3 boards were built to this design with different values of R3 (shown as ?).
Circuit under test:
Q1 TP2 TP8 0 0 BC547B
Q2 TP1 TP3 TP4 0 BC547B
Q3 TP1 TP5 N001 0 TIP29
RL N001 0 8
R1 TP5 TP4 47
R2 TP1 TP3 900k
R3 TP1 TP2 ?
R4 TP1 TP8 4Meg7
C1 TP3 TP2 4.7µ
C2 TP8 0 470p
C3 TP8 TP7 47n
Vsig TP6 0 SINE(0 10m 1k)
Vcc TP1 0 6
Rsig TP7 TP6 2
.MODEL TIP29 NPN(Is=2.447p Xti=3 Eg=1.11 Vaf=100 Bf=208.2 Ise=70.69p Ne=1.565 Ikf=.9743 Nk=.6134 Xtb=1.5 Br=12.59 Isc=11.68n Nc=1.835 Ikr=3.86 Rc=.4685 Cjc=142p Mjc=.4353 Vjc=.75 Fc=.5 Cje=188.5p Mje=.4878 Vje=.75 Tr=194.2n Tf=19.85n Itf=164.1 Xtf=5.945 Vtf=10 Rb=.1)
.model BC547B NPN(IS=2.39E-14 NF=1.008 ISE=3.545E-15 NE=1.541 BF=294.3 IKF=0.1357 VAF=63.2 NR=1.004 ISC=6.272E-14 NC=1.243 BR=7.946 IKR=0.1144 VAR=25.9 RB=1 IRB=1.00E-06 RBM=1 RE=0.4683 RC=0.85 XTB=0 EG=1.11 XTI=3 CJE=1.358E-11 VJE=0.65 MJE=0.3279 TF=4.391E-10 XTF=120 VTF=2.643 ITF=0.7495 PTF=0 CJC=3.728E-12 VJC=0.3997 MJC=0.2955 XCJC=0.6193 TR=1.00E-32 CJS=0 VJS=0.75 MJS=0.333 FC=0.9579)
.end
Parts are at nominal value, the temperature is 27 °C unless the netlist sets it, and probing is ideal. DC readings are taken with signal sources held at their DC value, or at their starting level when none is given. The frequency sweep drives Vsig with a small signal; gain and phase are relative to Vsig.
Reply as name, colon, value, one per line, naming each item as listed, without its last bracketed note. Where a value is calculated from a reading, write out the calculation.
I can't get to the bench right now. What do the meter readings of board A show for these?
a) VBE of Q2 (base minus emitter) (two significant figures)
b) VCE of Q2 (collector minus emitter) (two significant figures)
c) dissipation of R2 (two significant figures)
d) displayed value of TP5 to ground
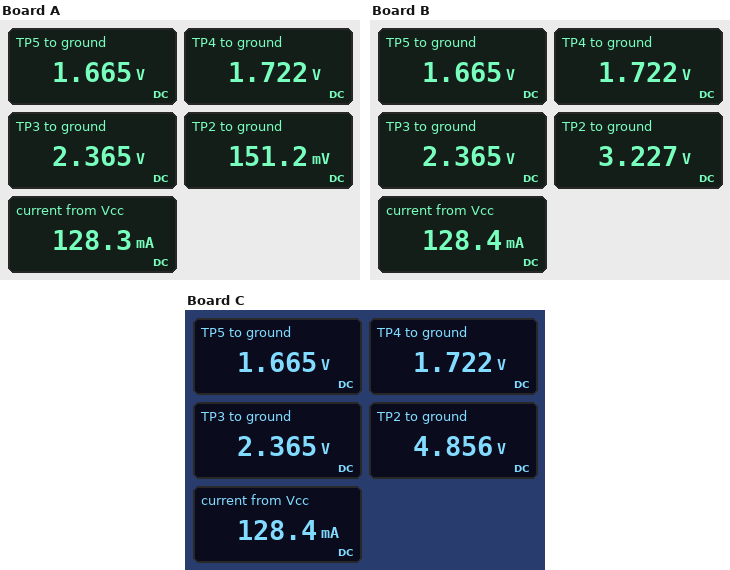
VBE of Q2 (base minus emitter): 2.365 V - 1.722 V = 640 mV
VCE of Q2 (collector minus emitter): 6 V - 1.722 V = 4.3 V
dissipation of R2: (6 V - 2.365 V)^2 / 900 kΩ = 15 µW
displayed value of TP5 to ground: 1.665 V
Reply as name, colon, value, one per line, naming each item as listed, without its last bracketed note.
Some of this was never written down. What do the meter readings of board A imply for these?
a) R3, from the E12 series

R3, from the E12 series: 22 kΩ
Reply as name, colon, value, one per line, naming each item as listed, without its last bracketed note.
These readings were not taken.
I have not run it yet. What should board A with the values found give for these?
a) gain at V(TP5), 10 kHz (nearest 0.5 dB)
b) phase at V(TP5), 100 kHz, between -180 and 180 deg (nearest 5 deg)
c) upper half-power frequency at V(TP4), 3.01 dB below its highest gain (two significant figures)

gain at V(TP5), 10 kHz: 39.0 dB
phase at V(TP5), 100 kHz, between -180 and 180 deg: 165 deg
upper half-power frequency at V(TP4), 3.01 dB below its highest gain: 470 kHz
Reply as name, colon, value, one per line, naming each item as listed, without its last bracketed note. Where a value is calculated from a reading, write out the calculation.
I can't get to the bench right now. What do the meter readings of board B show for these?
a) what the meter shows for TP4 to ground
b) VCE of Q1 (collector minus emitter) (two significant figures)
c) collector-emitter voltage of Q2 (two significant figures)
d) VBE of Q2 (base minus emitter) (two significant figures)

what the meter shows for TP4 to ground: 1.722 V
VCE of Q1 (collector minus emitter): 3.227 V = 3.2 V
collector-emitter voltage of Q2: 6 V - 1.722 V = 4.3 V
VBE of Q2 (base minus emitter): 2.365 V - 1.722 V = 640 mV
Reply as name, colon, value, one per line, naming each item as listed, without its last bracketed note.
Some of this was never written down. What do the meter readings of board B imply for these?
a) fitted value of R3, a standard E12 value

fitted value of R3, a standard E12 value: 8.2 kΩ
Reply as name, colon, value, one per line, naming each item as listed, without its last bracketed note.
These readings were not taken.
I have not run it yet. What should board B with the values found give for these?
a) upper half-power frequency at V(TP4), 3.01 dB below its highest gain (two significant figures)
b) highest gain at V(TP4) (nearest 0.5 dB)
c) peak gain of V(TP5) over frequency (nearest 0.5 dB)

upper half-power frequency at V(TP4), 3.01 dB below its highest gain: 1.1 MHz
highest gain at V(TP4): 39.5 dB
peak gain of V(TP5) over frequency: 39.0 dB
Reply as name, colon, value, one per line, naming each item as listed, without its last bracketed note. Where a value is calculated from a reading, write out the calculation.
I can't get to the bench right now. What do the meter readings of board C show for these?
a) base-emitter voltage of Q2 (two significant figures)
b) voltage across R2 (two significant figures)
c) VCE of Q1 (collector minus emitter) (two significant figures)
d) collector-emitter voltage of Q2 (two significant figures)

base-emitter voltage of Q2: 2.365 V - 1.722 V = 640 mV
voltage across R2: 6 V - 2.365 V = 3.6 V
VCE of Q1 (collector minus emitter): 4.856 V = 4.9 V
collector-emitter voltage of Q2: 6 V - 1.722 V = 4.3 V
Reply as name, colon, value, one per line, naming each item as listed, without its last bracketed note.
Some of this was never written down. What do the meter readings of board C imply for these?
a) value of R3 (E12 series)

value of R3: 3.3 kΩ
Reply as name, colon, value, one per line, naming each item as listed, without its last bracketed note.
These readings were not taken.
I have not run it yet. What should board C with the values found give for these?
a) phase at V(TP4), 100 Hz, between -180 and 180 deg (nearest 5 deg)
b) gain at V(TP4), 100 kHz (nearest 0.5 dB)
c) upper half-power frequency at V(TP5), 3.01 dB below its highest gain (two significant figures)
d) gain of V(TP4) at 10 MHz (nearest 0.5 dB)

phase at V(TP4), 100 Hz, between -180 and 180 deg: -125 deg
gain at V(TP4), 100 kHz: 32.0 dB
upper half-power frequency at V(TP5), 3.01 dB below its highest gain: 980 kHz
gain of V(TP4) at 10 MHz: 16.0 dB
